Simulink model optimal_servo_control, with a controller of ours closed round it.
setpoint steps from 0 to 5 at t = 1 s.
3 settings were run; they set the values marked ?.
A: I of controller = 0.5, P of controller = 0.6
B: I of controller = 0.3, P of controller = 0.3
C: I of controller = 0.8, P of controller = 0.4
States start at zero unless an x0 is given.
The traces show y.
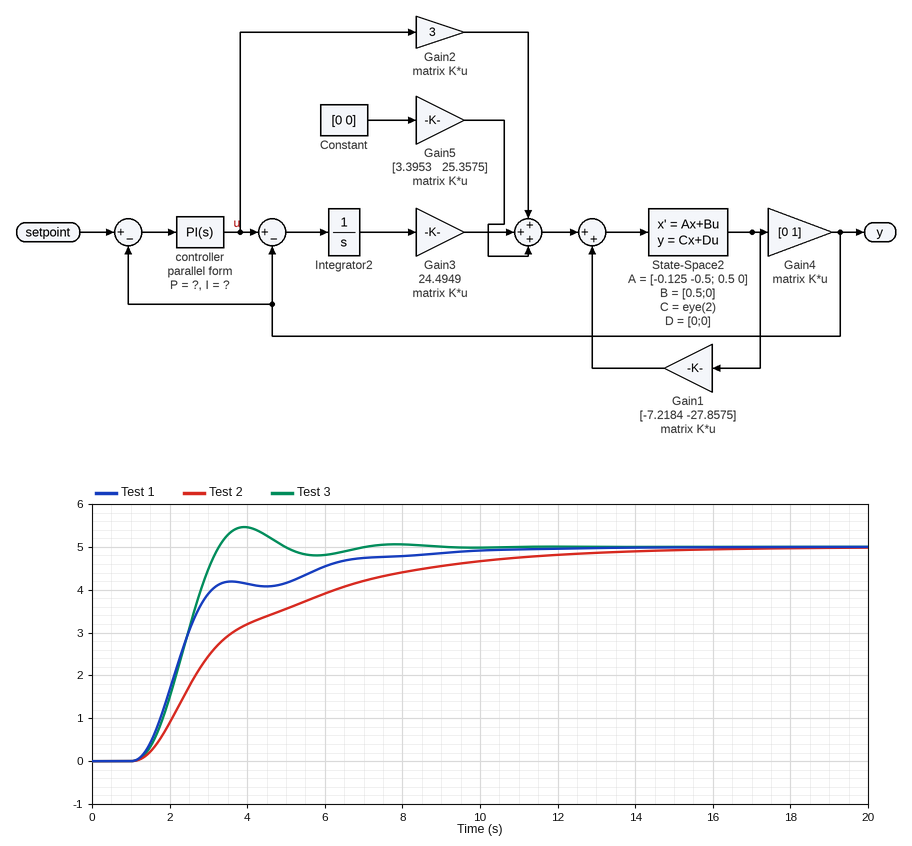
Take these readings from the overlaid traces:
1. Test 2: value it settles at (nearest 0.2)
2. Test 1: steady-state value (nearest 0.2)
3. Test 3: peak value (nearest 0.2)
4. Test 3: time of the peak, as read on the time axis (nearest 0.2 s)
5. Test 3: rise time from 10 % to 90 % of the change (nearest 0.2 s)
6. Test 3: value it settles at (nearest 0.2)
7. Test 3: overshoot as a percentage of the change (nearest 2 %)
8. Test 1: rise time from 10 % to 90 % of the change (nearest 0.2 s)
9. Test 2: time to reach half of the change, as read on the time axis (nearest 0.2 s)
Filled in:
5.0
5.0
5.4
4.0 s
1.4 s
5.0
10 %
4.4 s
3.0 s
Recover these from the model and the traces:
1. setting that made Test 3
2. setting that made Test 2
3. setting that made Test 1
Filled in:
C
B
A
